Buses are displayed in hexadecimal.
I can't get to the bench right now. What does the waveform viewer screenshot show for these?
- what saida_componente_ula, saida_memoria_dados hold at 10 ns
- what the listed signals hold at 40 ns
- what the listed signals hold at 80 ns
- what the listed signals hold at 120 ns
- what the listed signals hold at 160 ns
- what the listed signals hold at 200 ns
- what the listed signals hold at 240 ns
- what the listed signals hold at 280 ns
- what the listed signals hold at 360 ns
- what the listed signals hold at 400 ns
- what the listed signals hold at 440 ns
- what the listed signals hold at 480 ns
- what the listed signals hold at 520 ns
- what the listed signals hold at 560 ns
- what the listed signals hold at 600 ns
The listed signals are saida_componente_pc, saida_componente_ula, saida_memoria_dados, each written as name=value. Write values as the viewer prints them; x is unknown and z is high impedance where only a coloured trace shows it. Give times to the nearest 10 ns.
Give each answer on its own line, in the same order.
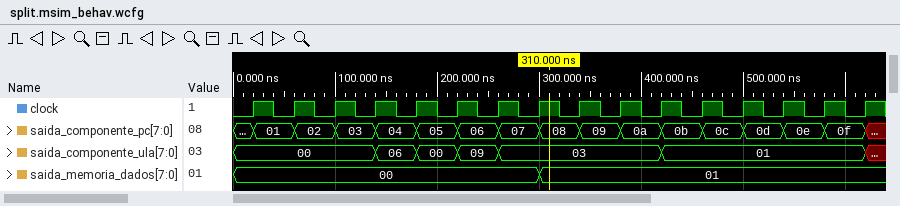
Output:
saida_componente_ula=00, saida_memoria_dados=00
saida_componente_pc=01, saida_componente_ula=00, saida_memoria_dados=00
saida_componente_pc=02, saida_componente_ula=00, saida_memoria_dados=00
saida_componente_pc=03, saida_componente_ula=00, saida_memoria_dados=00
saida_componente_pc=04, saida_componente_ula=06, saida_memoria_dados=00
saida_componente_pc=05, saida_componente_ula=00, saida_memoria_dados=00
saida_componente_pc=06, saida_componente_ula=09, saida_memoria_dados=00
saida_componente_pc=07, saida_componente_ula=03, saida_memoria_dados=00
saida_componente_pc=09, saida_componente_ula=03, saida_memoria_dados=01
saida_componente_pc=0a, saida_componente_ula=03, saida_memoria_dados=01
saida_componente_pc=0b, saida_componente_ula=01, saida_memoria_dados=01
saida_componente_pc=0c, saida_componente_ula=01, saida_memoria_dados=01
saida_componente_pc=0d, saida_componente_ula=01, saida_memoria_dados=01
saida_componente_pc=0e, saida_componente_ula=01, saida_memoria_dados=01
saida_componente_pc=0f, saida_componente_ula=01, saida_memoria_dados=01
